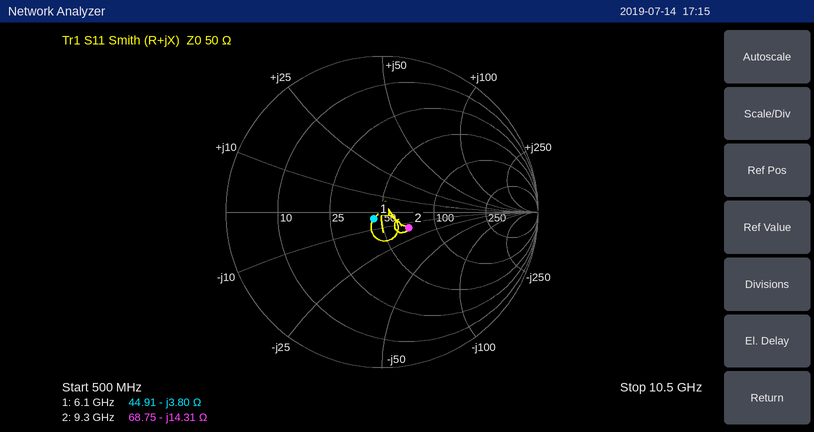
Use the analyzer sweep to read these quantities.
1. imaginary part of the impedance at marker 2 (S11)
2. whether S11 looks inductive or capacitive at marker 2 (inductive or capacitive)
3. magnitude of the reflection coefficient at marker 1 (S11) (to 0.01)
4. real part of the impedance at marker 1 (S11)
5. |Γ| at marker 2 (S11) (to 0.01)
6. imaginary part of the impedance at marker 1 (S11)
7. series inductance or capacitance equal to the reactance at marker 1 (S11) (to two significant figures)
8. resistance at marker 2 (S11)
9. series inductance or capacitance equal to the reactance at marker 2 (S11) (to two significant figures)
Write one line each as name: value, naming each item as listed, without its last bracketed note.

imaginary part of the impedance at marker 2: -14.31 Ω
whether S11 looks inductive or capacitive at marker 2: capacitive
magnitude of the reflection coefficient at marker 1 (S11): 0.07
real part of the impedance at marker 1: 44.91 Ω
|Γ| at marker 2 (S11): 0.20
imaginary part of the impedance at marker 1: -3.80 Ω
series inductance or capacitance equal to the reactance at marker 1 (S11): 6.9 pF
resistance at marker 2: 68.75 Ω
series inductance or capacitance equal to the reactance at marker 2 (S11): 1.2 pF
